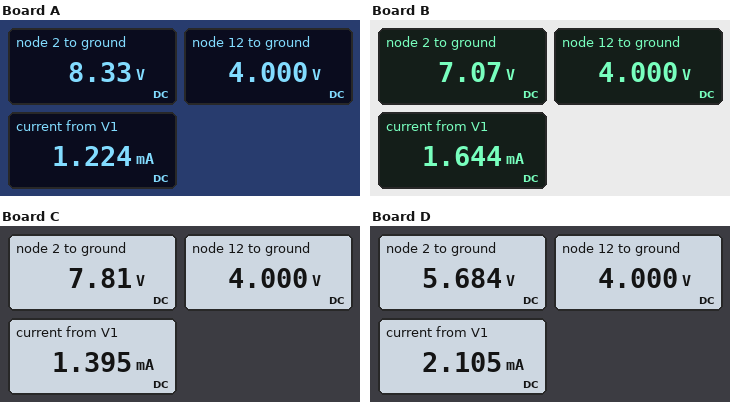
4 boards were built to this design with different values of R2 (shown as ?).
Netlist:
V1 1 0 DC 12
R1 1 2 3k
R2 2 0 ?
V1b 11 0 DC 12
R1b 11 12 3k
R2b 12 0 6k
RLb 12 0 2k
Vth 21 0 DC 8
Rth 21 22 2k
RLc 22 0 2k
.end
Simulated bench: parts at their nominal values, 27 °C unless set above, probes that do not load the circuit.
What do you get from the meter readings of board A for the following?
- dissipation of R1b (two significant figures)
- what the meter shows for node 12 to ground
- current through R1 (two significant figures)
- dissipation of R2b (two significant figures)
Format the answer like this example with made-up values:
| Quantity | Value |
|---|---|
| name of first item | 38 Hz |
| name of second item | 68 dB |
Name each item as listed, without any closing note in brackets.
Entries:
| Quantity | Value |
|---|---|
| dissipation of R1b | 21 mW |
| what the meter shows for node 12 to ground | 4.000 V |
| current through R1 | 1.2 mA |
| dissipation of R2b | 2.7 mW |
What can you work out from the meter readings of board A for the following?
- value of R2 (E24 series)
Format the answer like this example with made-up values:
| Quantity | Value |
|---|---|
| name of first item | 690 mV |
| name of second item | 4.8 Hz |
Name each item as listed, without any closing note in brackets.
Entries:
| Quantity | Value |
|---|---|
| value of R2 | 6.8 kΩ |
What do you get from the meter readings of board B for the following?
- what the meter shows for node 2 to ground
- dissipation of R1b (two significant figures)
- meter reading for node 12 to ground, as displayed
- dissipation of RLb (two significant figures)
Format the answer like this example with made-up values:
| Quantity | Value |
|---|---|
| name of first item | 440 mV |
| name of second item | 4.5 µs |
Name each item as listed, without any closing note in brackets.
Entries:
| Quantity | Value |
|---|---|
| what the meter shows for node 2 to ground | 7.07 V |
| dissipation of R1b | 21 mW |
| meter reading for node 12 to ground, as displayed | 4.000 V |
| dissipation of RLb | 8.0 mW |
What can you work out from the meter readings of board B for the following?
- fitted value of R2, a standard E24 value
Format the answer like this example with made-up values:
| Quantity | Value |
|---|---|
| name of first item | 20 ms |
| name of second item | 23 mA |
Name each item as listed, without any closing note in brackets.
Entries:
| Quantity | Value |
|---|---|
| fitted value of R2, a standard E24 value | 4.3 kΩ |
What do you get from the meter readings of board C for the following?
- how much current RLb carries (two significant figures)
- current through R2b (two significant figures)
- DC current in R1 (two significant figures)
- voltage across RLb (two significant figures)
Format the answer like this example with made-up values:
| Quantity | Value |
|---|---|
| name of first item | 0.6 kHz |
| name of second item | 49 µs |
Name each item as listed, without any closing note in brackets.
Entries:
| Quantity | Value |
|---|---|
| how much current RLb carries | 2.0 mA |
| current through R2b | 670 µA |
| DC current in R1 | 1.4 mA |
| voltage across RLb | 4.0 V |
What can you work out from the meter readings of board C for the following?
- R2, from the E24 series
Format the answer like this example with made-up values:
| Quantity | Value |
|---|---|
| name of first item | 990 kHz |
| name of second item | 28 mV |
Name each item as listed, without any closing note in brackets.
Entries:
| Quantity | Value |
|---|---|
| R2, from the E24 series | 5.6 kΩ |
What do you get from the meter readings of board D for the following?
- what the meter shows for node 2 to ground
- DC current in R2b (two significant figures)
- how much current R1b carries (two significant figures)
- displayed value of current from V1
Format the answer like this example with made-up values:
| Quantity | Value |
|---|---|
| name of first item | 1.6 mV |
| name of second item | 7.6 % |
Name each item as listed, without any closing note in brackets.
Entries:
| Quantity | Value |
|---|---|
| what the meter shows for node 2 to ground | 5.684 V |
| DC current in R2b | 670 µA |
| how much current R1b carries | 2.7 mA |
| displayed value of current from V1 | 2.105 mA |
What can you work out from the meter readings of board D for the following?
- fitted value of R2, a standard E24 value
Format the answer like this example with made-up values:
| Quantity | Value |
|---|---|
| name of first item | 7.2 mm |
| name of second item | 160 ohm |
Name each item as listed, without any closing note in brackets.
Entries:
| Quantity | Value |
|---|---|
| fitted value of R2, a standard E24 value | 2.7 kΩ |
